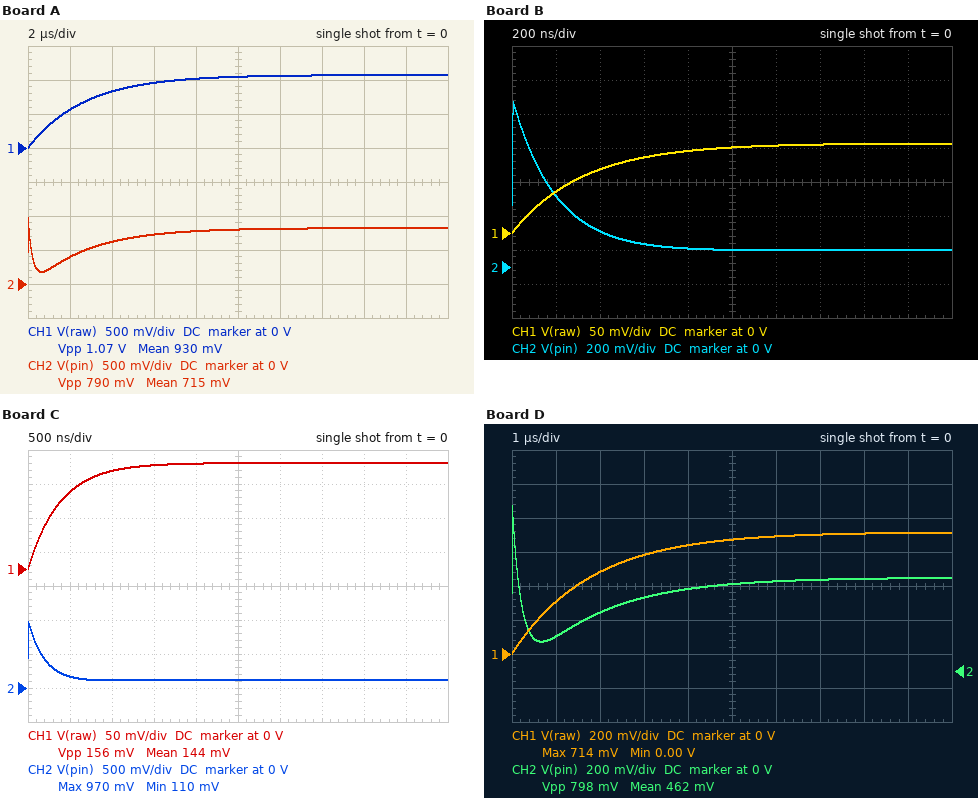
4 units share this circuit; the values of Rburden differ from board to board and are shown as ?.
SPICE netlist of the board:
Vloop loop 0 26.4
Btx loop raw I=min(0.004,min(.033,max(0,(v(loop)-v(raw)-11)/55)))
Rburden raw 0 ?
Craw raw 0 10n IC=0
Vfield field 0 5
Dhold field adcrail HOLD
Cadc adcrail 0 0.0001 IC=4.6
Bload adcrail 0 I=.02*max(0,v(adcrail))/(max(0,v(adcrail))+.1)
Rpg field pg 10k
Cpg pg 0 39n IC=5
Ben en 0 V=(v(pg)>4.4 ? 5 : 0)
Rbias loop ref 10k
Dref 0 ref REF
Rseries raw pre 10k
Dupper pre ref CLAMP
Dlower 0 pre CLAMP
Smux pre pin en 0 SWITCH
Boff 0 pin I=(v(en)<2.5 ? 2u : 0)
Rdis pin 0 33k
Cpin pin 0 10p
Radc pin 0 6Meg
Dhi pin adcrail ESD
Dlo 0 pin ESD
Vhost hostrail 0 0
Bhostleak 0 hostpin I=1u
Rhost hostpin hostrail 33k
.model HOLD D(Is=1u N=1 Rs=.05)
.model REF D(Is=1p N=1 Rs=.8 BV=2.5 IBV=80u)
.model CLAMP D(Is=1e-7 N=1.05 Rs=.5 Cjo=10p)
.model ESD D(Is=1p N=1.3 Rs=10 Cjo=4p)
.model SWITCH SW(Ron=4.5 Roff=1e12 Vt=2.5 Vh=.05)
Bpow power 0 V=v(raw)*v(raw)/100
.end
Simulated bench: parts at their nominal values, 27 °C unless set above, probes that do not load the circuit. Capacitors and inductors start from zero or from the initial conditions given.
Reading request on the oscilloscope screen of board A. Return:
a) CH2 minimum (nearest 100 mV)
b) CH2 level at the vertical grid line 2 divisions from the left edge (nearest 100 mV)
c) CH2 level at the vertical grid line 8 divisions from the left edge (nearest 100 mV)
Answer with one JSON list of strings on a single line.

["200 mV", "600 mV", "800 mV"]
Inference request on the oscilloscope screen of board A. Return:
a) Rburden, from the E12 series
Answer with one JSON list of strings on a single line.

["270 Ω"]
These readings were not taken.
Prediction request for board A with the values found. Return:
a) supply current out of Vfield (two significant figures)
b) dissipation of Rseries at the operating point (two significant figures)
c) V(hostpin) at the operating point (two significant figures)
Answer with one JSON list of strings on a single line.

["20 mA", "6.3 µW", "33 mV"]
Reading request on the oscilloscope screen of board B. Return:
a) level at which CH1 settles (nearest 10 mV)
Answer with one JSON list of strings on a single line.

["130 mV"]
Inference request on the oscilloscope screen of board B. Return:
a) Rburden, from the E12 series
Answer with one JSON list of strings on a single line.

["33 Ω"]
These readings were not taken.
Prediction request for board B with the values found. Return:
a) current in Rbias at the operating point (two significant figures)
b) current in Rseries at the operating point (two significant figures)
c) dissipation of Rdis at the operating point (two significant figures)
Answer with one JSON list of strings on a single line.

["2.4 mA", "3.1 µA", "310 nW"]
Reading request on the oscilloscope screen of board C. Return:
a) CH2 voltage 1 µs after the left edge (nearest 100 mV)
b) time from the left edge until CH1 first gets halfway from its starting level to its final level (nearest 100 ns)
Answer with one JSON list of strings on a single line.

["100 mV", "300 ns"]
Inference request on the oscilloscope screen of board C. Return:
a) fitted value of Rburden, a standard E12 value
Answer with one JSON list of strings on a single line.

["39 Ω"]
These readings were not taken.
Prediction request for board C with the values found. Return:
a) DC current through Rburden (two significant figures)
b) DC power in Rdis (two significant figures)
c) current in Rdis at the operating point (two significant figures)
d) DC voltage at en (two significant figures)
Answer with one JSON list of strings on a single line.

["4.0 mA", "430 nW", "3.6 µA", "5.0 V"]
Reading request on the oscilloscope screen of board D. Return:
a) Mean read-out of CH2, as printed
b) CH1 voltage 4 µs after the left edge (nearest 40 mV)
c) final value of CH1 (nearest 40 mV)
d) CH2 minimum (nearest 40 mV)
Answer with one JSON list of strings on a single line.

["462 mV", "640 mV", "720 mV", "160 mV"]
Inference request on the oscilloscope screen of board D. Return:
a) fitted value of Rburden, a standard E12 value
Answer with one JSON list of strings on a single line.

["180 Ω"]
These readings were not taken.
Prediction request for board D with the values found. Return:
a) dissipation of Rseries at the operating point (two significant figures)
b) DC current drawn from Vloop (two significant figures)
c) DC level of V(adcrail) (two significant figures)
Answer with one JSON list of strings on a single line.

["2.8 µW", "6.4 mA", "4.7 V"]
